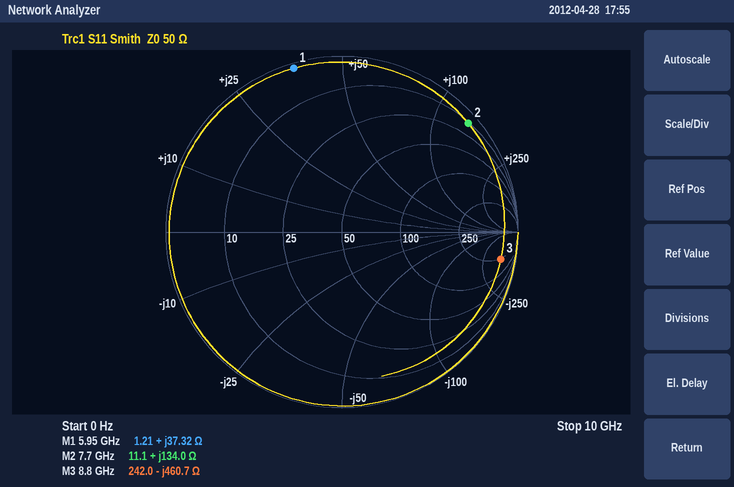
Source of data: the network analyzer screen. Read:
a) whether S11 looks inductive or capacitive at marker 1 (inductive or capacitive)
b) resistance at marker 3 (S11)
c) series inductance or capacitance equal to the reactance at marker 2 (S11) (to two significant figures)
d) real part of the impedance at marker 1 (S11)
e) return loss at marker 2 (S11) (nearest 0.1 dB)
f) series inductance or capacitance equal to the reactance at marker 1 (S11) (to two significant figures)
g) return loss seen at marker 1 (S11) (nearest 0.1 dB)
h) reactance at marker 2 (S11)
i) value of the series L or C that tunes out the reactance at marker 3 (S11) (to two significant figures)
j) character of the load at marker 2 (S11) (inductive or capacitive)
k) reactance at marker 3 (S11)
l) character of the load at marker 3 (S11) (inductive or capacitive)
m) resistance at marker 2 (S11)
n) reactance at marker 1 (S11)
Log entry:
inductive
242.0 Ω
2.8 nH
1.21 Ω
0.5 dB
1.00 nH
0.3 dB
+134.0 Ω
8.3 nH
inductive
-460.7 Ω
capacitive
11.1 Ω
+37.32 Ω
